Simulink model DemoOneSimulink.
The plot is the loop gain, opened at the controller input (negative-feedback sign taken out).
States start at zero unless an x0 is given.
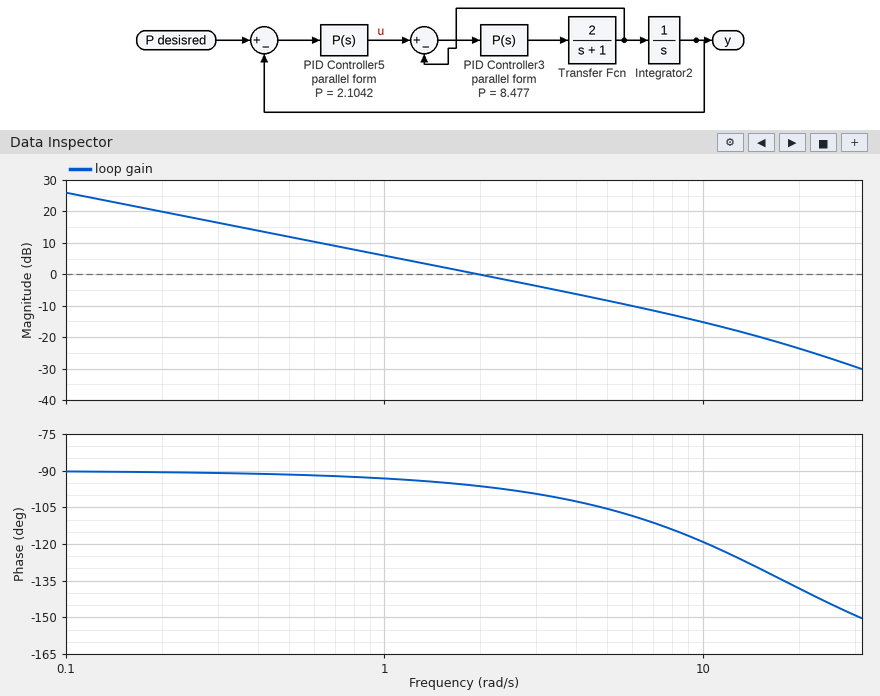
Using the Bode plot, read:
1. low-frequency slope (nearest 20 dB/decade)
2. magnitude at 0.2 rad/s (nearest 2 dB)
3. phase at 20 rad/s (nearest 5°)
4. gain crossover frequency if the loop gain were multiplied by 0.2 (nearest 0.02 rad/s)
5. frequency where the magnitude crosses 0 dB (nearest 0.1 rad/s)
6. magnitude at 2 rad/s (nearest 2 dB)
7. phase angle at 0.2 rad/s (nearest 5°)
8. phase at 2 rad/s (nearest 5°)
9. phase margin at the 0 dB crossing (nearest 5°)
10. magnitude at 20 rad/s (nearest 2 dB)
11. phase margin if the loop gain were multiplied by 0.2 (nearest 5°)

-20 dB/decade
20 dB
-140°
0.40 rad/s
2.0 rad/s
0 dB
-90°
-95°
85°
-24 dB
90°
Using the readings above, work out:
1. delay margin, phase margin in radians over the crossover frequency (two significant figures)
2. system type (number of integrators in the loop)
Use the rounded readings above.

0.74 s
1
